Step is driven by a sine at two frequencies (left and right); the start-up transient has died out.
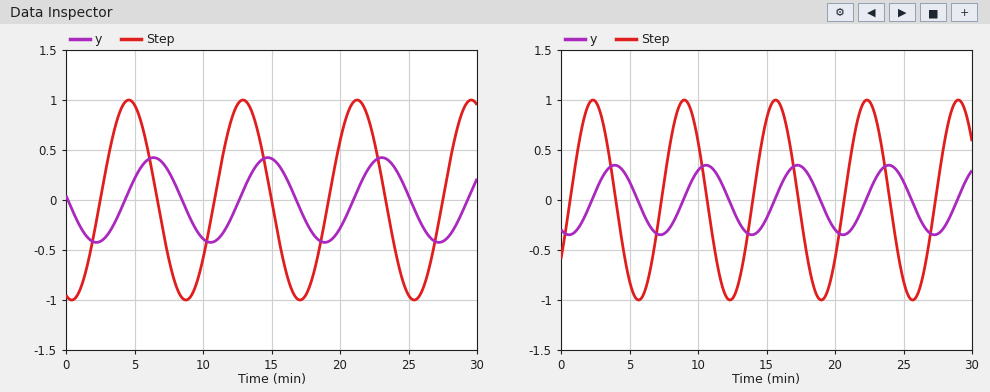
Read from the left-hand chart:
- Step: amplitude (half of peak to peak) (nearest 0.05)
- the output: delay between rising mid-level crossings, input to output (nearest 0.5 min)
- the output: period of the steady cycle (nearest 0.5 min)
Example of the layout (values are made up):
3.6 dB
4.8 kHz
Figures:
1.00
2.0 min
8.5 min
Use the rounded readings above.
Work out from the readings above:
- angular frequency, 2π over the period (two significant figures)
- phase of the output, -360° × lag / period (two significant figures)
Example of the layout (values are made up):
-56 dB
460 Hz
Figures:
0.74 rad/min
-85°
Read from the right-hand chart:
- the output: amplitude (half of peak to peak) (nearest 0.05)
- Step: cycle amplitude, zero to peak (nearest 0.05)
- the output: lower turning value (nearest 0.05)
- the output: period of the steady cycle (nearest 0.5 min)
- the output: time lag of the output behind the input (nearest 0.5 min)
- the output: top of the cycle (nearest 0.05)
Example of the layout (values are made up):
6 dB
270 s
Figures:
0.35
1.00
-0.35
6.5 min
1.5 min
0.35
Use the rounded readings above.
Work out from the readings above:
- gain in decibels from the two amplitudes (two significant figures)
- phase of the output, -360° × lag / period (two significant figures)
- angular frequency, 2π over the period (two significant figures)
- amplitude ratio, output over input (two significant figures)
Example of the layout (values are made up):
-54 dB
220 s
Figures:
-9.1 dB
-83°
0.97 rad/min
0.35
